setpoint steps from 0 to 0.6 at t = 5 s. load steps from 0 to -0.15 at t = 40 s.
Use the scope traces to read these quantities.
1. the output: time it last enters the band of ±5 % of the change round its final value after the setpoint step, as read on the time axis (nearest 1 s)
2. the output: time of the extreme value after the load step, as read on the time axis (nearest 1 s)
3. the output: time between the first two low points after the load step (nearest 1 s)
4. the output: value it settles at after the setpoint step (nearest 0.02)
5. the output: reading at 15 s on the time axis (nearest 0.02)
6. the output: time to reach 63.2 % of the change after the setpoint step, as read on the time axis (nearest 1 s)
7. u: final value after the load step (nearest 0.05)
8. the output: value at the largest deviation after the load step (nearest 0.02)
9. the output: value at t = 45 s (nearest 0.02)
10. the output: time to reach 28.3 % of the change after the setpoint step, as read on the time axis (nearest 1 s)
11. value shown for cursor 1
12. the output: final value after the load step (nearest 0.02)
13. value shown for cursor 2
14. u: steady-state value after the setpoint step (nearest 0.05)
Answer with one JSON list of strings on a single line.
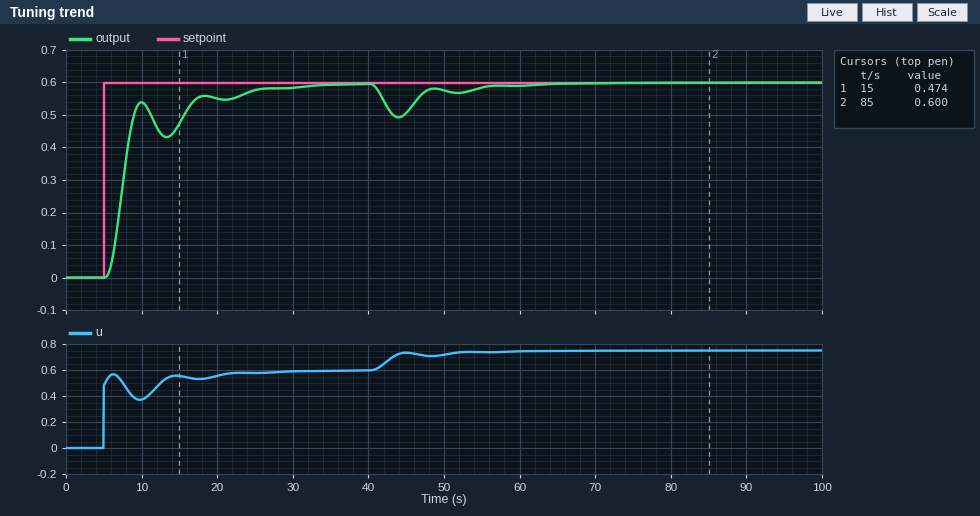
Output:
["24 s", "44 s", "8 s", "0.60", "0.48", "8 s", "0.75", "0.50", "0.50", "7 s", "0.474", "0.60", "0.600", "0.60"]
